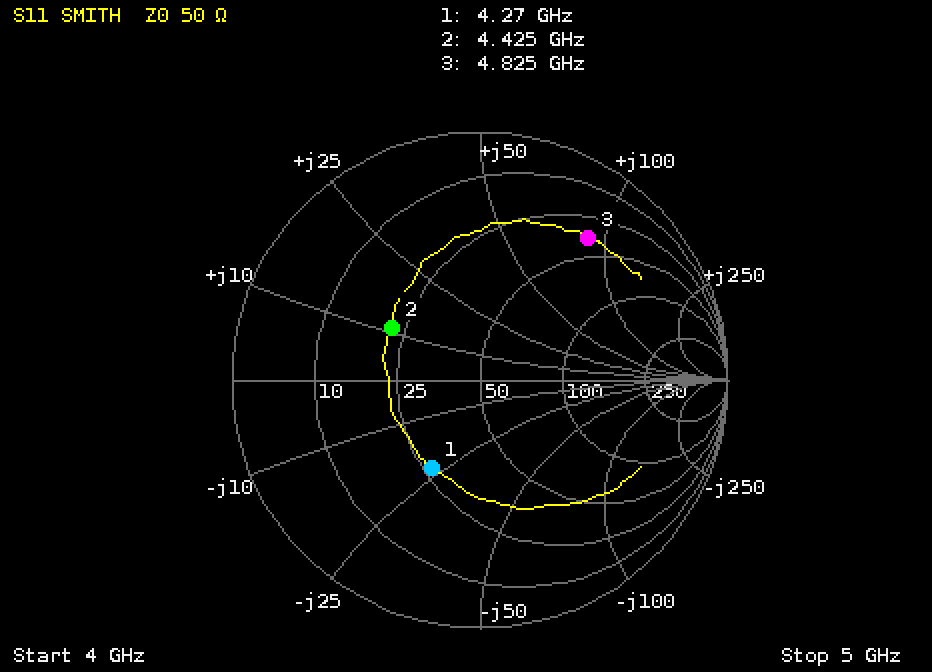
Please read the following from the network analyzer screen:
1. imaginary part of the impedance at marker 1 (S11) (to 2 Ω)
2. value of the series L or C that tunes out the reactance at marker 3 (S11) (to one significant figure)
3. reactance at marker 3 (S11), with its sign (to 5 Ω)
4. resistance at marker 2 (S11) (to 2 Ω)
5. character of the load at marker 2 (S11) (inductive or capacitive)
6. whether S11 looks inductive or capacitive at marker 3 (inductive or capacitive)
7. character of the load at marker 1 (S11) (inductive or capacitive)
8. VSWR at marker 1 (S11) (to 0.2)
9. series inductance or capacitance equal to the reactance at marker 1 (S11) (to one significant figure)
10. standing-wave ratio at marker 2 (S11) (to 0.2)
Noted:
-22 Ω
400 fF
+90 Ω
22 Ω
inductive
inductive
capacitive
2.4
2 pF
2.4
